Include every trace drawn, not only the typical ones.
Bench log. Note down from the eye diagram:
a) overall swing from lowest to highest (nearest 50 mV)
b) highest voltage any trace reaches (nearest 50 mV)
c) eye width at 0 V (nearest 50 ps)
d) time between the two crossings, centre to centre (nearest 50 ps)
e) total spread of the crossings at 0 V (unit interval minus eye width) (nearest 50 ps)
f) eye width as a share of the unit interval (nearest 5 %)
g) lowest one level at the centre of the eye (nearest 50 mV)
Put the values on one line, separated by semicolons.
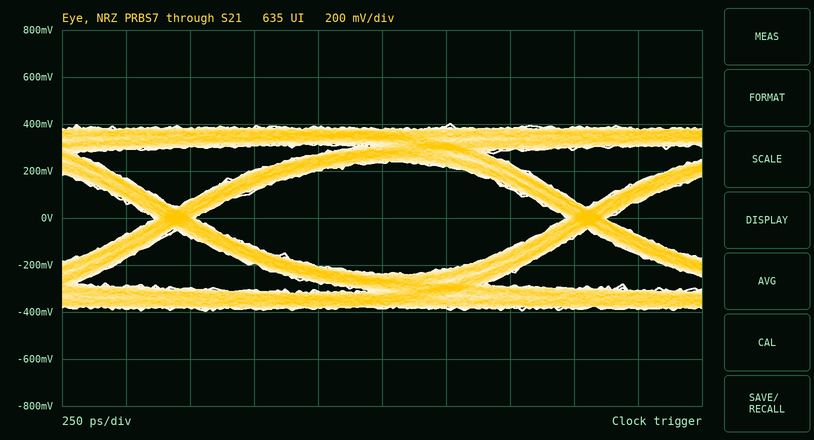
800 mV; 400 mV; 1.45 ns; 1.60 ns; 150 ps; 90 %; 250 mV
